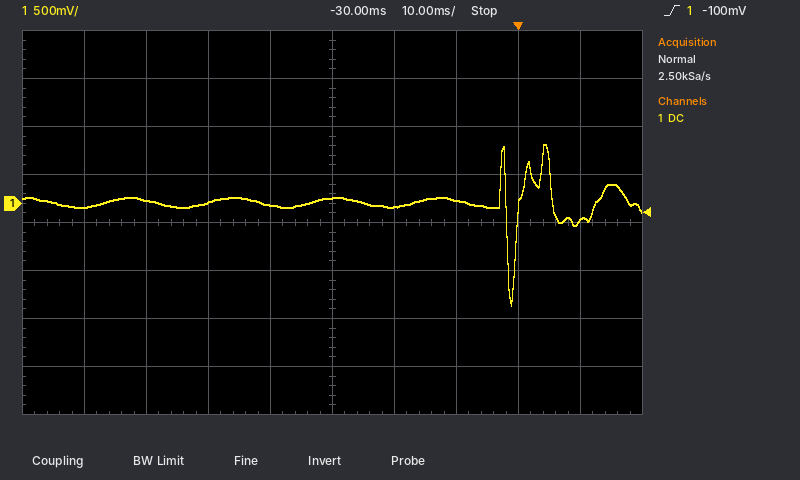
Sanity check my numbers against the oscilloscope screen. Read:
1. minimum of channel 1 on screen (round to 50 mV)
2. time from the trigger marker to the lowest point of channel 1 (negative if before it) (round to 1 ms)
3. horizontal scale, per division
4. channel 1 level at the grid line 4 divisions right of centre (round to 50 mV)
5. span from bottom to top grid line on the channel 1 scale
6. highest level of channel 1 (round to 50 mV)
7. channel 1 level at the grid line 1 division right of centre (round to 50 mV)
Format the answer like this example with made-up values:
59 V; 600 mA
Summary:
-1.05 V; -1 ms; 10 ms; -200 mV; 4 V; 600 mV; -50 mV
